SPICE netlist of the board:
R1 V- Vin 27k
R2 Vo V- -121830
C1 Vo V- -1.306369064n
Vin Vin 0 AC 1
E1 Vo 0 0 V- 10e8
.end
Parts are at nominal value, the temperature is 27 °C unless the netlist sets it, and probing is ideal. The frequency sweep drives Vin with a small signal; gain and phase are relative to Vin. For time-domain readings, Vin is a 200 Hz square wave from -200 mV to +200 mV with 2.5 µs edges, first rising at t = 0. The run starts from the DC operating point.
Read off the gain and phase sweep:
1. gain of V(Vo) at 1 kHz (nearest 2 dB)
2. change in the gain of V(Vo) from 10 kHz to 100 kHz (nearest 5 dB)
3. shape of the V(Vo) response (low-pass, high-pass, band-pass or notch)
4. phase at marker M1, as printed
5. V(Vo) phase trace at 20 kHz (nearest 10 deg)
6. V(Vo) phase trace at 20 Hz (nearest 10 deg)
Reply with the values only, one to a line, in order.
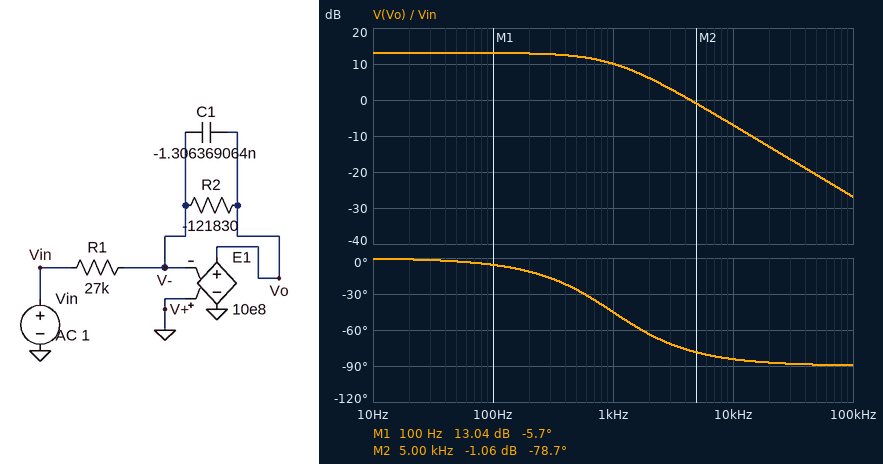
10 dB
-20 dB
low-pass
-5.7 deg
-90 deg
0 deg
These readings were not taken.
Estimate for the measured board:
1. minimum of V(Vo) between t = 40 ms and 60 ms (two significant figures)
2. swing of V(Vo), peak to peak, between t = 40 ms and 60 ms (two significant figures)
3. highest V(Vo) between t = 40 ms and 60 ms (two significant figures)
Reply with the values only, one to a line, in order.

-900 mV
1.8 V
900 mV
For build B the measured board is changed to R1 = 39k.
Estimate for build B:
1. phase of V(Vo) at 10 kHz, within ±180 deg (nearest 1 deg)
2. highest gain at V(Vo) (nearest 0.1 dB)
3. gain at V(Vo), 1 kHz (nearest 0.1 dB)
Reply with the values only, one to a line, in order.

-84 deg
9.9 dB
6.9 dB
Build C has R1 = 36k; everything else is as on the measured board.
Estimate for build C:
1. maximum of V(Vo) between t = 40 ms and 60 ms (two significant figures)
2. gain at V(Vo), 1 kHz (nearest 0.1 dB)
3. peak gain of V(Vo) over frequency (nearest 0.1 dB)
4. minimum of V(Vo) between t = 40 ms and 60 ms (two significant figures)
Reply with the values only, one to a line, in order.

680 mV
7.6 dB
10.6 dB
-680 mV
